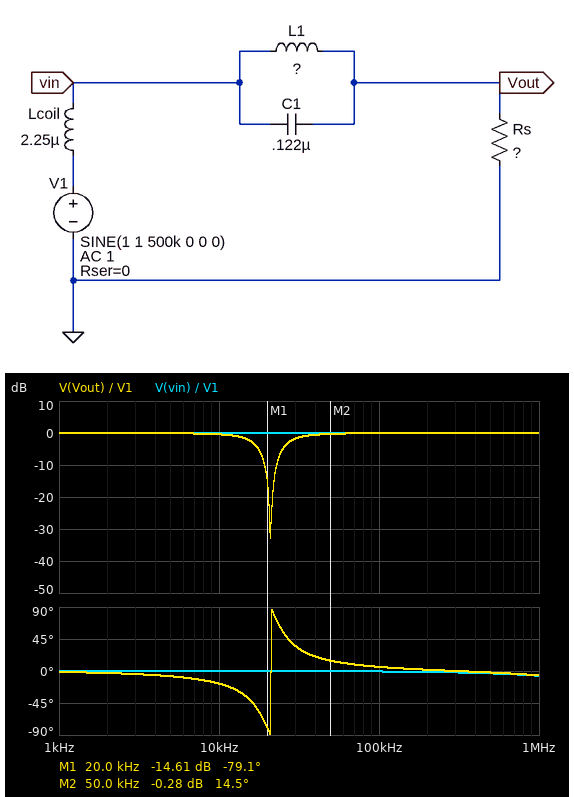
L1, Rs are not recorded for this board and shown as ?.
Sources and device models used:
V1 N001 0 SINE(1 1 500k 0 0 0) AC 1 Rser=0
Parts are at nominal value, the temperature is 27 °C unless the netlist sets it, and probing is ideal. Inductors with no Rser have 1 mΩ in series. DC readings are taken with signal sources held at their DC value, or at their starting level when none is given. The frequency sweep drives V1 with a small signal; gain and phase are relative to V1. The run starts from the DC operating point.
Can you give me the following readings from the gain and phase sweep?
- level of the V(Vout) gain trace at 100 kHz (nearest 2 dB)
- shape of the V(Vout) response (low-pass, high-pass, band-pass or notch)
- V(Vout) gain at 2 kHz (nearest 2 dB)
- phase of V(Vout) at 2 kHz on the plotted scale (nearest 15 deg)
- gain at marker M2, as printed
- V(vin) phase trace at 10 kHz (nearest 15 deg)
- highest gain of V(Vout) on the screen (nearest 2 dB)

0 dB
notch
0 dB
0 deg
-0.28 dB
0 deg
0 dB
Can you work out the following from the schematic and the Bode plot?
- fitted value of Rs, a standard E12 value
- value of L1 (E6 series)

120 Ω
470 µH
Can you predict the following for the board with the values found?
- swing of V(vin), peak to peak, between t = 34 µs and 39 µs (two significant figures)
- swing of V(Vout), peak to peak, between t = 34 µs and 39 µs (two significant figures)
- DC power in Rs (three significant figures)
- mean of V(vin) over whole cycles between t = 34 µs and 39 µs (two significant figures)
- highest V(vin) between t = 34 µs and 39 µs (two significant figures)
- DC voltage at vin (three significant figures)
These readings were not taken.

2.0 V
2.0 V
8.33 mW
1.0 V
2.0 V
1.00 V
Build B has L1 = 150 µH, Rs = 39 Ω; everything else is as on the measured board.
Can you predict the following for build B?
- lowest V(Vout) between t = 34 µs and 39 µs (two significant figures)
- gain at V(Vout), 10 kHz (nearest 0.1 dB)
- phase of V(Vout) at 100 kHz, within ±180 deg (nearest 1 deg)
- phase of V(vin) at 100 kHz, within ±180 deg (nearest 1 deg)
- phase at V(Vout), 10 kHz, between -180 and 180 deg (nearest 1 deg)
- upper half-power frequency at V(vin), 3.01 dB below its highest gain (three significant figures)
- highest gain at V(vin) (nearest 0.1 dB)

6.5 mV
-0.3 dB
19 deg
-2 deg
-15 deg
2.73 MHz
0.1 dB
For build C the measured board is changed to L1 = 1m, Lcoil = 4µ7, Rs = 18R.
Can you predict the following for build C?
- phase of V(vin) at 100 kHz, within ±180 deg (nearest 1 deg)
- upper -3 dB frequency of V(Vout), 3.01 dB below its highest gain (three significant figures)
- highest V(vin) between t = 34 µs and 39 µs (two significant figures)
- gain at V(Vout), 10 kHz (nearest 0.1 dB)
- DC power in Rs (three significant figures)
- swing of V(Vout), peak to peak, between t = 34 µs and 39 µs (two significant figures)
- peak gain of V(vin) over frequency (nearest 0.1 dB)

-7 deg
675 kHz
1.8 V
-16.7 dB
55.5 mW
1.7 V
0.7 dB
